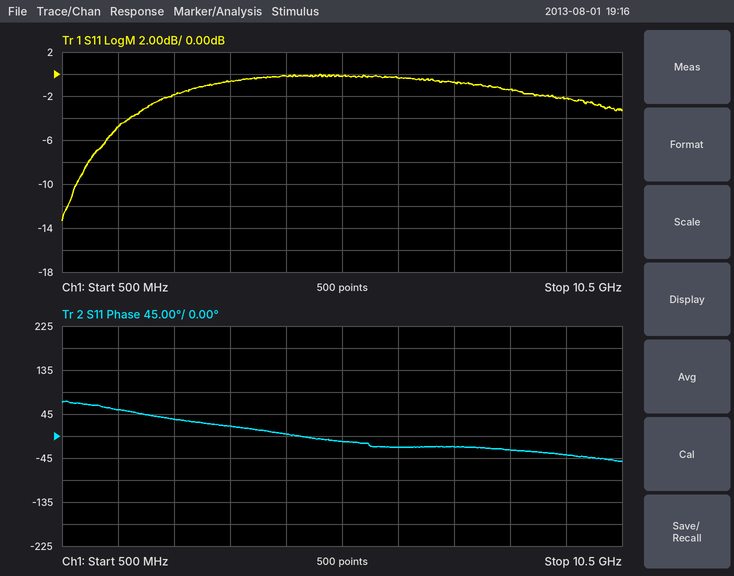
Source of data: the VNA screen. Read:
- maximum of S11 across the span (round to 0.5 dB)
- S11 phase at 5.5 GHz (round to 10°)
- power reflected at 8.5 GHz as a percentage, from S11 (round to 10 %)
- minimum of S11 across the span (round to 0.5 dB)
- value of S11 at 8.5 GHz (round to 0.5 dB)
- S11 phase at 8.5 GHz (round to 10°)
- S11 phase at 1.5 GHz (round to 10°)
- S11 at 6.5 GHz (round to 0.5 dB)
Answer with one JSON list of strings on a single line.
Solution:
["0.0 dB", "-10°", "70 %", "-13.5 dB", "-1.5 dB", "-30°", "50°", "-0.5 dB"]
